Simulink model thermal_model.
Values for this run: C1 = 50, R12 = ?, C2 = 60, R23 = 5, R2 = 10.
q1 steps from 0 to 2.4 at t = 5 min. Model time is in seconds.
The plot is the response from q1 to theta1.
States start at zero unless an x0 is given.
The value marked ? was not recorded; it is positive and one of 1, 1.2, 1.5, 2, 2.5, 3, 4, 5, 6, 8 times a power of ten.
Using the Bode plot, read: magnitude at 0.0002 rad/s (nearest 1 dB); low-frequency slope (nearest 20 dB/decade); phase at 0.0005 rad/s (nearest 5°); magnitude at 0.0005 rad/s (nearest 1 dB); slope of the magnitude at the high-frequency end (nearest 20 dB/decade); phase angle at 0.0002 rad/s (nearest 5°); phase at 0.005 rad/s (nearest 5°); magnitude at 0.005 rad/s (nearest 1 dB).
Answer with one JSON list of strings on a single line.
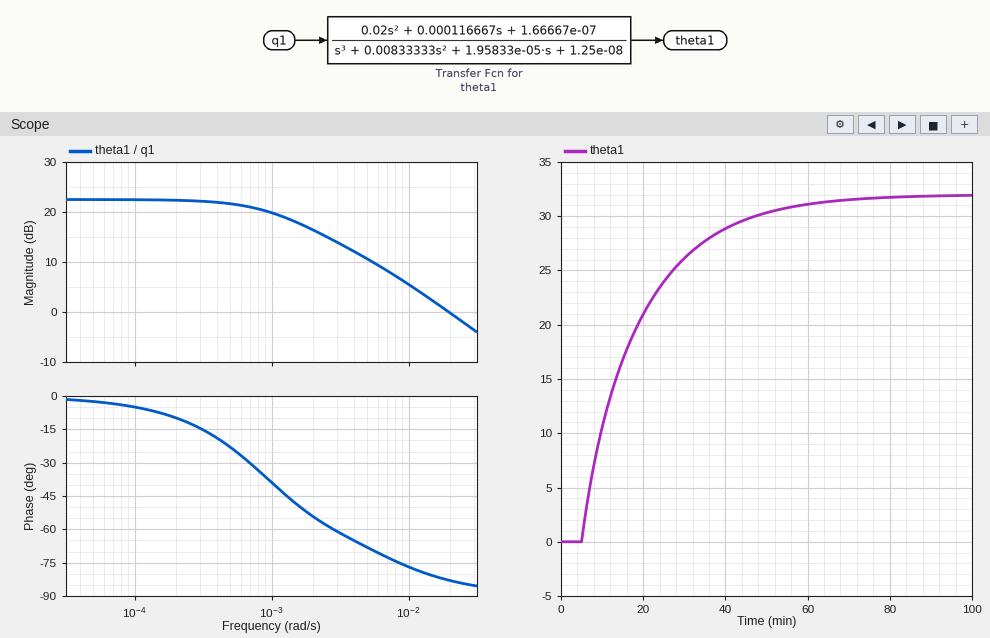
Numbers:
["22 dB", "0 dB/decade", "-25°", "22 dB", "-20 dB/decade", "-10°", "-70°", "11 dB"]
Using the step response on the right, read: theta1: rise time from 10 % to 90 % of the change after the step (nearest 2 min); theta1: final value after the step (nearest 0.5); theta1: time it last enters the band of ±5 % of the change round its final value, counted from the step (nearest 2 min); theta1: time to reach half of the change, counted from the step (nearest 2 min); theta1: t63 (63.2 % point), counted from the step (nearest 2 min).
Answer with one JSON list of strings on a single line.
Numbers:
["34 min", "32.0", "46 min", "10 min", "14 min"]
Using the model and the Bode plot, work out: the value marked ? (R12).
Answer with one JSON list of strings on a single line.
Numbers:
["8"]
